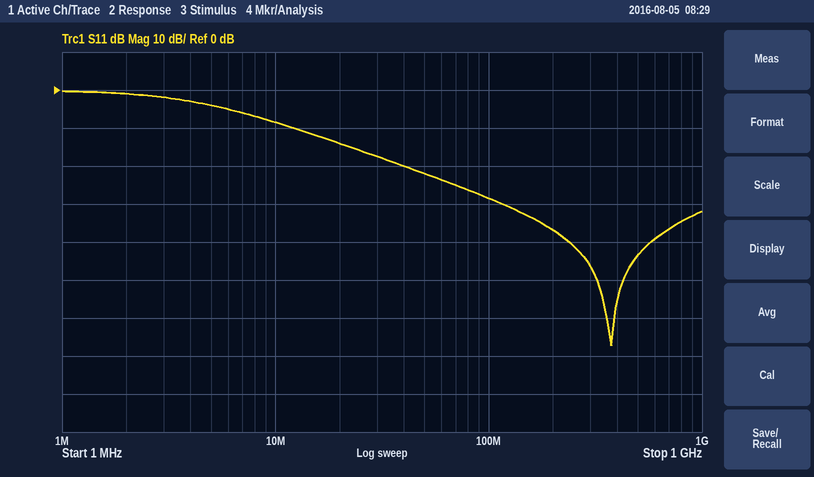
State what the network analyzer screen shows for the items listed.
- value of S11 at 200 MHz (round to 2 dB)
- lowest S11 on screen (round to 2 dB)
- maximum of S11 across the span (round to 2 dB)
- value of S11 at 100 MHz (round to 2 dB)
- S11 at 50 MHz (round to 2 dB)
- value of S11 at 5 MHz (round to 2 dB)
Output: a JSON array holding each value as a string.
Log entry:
["-36 dB", "-68 dB", "0 dB", "-28 dB", "-22 dB", "-4 dB"]
